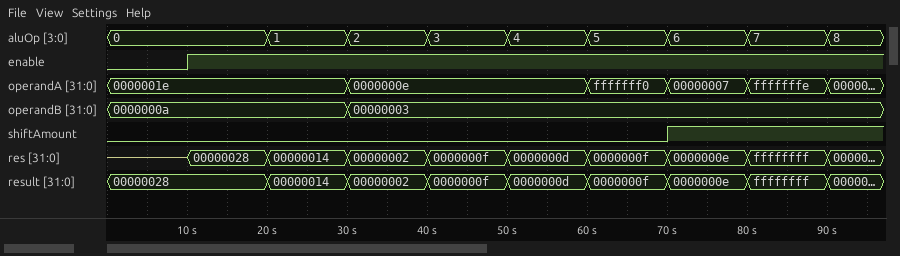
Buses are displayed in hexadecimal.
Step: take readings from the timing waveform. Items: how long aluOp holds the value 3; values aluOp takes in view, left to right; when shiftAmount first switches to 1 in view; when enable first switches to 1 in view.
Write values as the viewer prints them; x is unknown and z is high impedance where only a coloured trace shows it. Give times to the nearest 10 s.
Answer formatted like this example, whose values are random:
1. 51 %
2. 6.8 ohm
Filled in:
1. 10 s
2. 0, 1, 2, 3, 4, 5, 6, 7, 8
3. 70 s
4. 10 s
